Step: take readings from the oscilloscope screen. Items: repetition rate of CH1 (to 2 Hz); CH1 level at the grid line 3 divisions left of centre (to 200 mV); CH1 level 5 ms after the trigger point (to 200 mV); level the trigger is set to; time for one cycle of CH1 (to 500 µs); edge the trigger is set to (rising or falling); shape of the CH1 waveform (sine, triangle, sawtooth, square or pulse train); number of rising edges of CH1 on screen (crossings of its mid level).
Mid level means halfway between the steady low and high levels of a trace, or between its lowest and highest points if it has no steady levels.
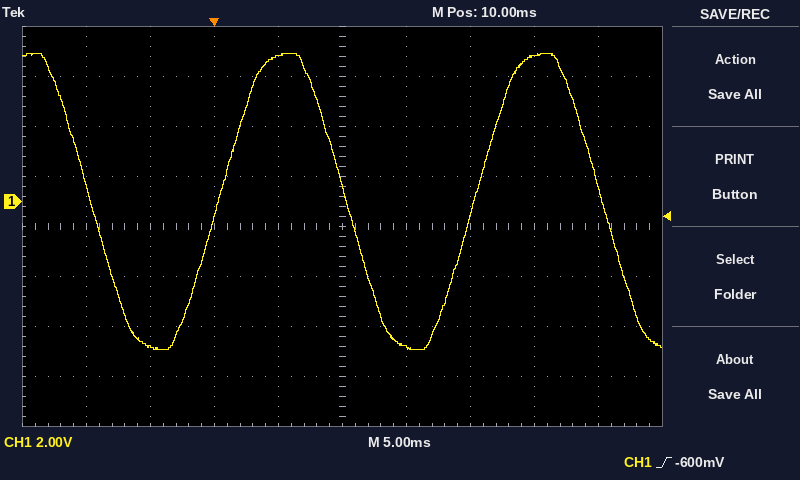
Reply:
50 Hz
-5.8 V
5.8 V
-600 mV
20.0 ms
rising
sine
2
